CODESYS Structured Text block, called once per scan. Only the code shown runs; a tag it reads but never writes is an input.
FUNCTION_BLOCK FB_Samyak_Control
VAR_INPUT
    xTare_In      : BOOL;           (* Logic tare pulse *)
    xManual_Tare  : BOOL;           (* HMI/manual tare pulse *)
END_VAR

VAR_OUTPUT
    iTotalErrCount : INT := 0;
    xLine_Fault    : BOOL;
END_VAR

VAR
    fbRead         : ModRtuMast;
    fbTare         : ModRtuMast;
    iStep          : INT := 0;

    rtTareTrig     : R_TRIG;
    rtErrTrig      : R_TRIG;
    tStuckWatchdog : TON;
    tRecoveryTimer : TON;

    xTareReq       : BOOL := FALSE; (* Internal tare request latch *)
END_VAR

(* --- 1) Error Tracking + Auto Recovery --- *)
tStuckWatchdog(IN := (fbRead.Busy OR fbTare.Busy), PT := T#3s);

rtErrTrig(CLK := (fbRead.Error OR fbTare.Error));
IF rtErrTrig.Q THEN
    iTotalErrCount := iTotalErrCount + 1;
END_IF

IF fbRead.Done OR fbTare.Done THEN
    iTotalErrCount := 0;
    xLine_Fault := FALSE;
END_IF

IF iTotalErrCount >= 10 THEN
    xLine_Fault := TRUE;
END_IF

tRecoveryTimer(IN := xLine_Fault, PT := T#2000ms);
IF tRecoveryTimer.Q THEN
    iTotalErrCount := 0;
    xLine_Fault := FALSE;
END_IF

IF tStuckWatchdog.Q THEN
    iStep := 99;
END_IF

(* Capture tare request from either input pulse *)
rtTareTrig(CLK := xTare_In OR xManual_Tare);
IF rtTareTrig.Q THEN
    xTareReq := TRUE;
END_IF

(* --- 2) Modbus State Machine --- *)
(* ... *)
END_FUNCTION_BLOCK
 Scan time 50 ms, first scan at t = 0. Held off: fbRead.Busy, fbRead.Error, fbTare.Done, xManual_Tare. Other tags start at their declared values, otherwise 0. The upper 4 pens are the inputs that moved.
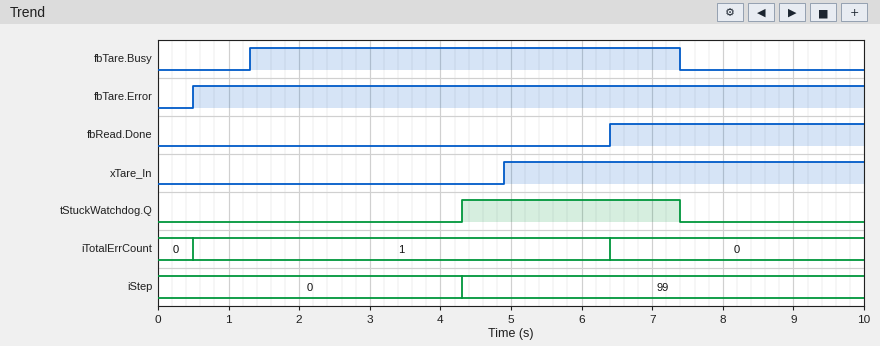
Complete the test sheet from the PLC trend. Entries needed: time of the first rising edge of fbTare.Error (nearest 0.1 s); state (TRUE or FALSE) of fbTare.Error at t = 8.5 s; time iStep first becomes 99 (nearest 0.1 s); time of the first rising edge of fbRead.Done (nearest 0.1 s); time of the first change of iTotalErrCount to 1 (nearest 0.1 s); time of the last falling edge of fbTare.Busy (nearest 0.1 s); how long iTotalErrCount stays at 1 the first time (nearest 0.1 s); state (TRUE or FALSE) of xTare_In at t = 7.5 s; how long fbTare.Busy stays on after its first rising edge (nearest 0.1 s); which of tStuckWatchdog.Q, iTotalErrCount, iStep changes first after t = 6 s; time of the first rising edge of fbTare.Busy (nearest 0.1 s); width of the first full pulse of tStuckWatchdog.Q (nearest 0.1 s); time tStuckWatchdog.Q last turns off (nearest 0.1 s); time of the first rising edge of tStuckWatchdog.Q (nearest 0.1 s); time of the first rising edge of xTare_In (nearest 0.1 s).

0.5 s
TRUE
4.3 s
6.4 s
0.5 s
7.4 s
5.9 s
TRUE
6.1 s
iTotalErrCount
1.3 s
3.1 s
7.4 s
4.3 s
4.9 s
